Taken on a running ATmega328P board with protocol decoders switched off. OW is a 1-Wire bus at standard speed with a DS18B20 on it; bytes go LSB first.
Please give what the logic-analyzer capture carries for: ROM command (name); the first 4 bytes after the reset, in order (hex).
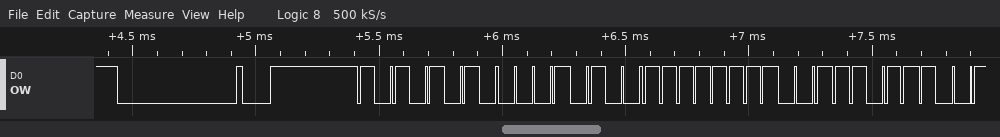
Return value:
Match ROM
55 28 FF DC
